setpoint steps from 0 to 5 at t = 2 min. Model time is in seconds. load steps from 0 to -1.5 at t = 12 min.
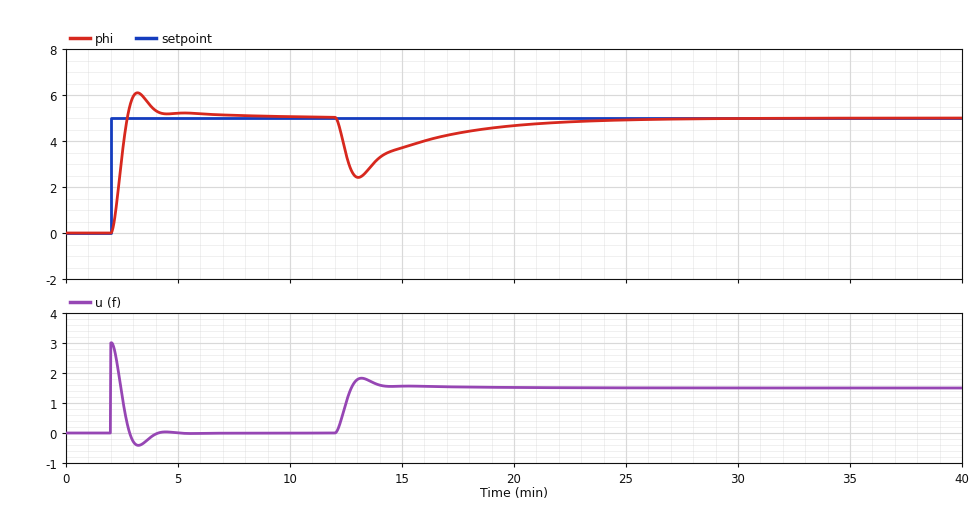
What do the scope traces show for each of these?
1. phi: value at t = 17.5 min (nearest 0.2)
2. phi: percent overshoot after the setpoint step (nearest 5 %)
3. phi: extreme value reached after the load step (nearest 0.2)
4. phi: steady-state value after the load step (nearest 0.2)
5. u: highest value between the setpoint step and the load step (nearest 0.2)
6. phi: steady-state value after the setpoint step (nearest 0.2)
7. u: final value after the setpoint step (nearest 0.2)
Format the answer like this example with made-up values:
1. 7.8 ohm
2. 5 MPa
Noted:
1. 4.4
2. 20 %
3. 2.4
4. 5.0
5. 3.0
6. 5.0
7. 0.0
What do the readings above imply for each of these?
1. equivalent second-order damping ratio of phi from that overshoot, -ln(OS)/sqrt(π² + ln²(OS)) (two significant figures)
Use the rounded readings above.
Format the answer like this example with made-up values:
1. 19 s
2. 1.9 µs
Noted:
1. 0.46
